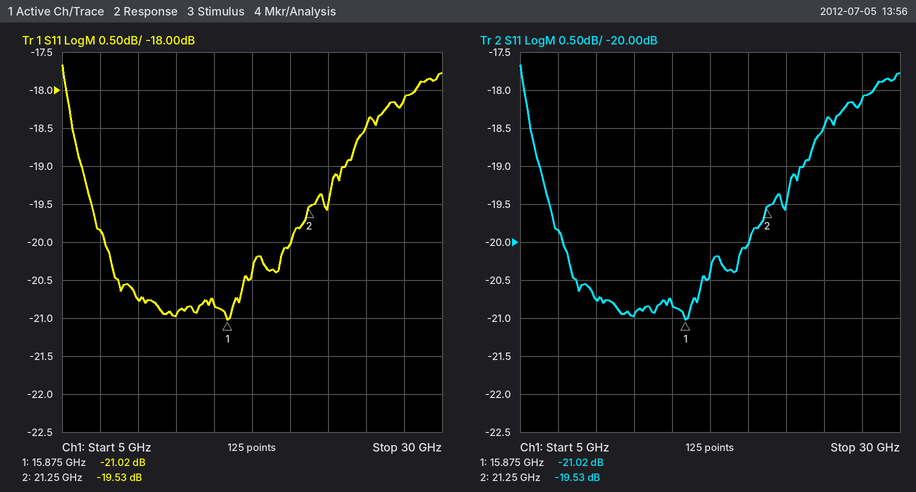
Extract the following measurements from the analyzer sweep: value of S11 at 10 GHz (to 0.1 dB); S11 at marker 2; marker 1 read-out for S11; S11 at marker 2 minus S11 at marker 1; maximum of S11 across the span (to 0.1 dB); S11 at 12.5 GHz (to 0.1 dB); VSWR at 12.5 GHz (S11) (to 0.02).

-20.8 dB
-19.53 dB
-21.02 dB
1.49 dB
-17.7 dB
-21.0 dB
1.20
